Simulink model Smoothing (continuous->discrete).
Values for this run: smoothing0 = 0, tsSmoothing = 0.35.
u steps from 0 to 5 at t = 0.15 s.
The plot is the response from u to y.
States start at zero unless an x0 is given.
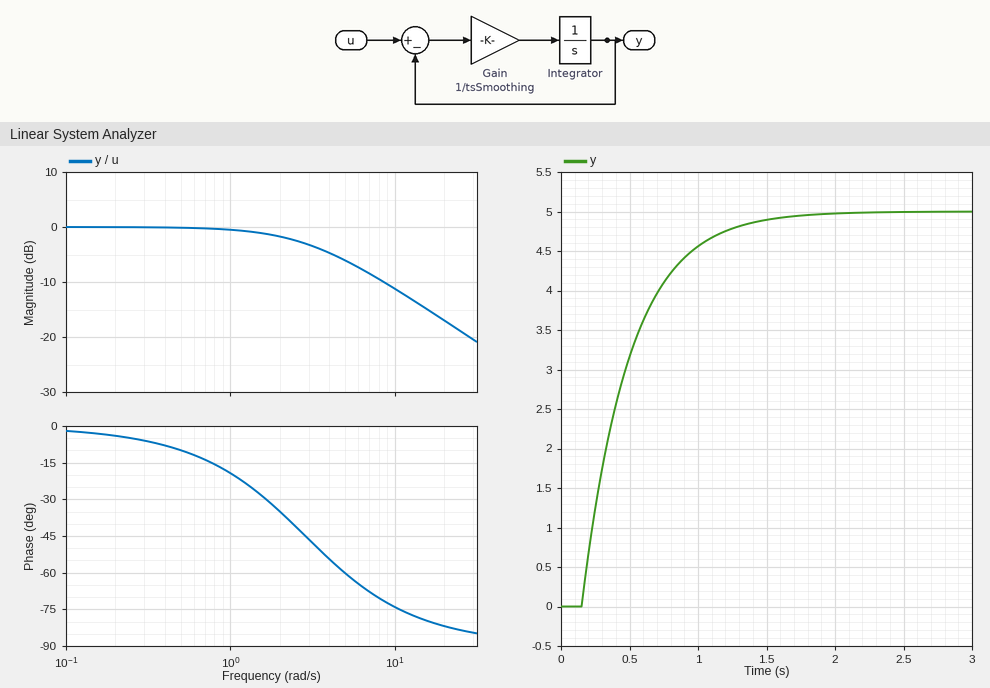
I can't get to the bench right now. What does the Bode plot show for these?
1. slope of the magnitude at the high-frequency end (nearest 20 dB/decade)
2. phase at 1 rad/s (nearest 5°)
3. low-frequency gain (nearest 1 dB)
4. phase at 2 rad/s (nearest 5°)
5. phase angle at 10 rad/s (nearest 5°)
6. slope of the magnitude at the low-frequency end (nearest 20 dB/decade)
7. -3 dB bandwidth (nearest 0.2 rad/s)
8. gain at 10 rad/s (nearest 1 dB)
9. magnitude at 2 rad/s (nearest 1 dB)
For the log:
-20 dB/decade
-20°
0 dB
-35°
-75°
0 dB/decade
2.8 rad/s
-11 dB
-2 dB
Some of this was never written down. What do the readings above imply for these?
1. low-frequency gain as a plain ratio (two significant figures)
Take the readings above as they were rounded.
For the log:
1.0
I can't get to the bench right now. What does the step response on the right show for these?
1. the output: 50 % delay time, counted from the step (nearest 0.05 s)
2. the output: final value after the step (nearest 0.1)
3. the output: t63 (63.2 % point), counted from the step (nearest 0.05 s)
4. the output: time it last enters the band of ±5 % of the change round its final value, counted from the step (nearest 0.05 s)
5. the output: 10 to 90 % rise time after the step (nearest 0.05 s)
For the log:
0.25 s
5.0
0.35 s
1.05 s
0.75 s
